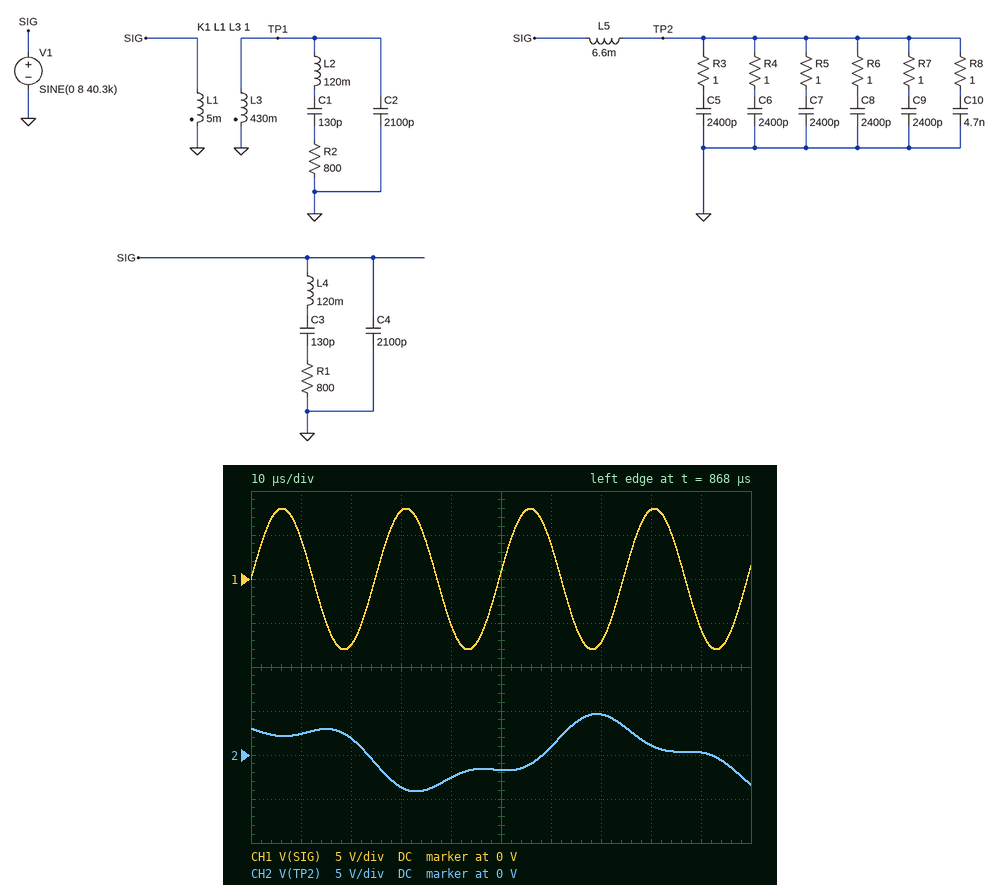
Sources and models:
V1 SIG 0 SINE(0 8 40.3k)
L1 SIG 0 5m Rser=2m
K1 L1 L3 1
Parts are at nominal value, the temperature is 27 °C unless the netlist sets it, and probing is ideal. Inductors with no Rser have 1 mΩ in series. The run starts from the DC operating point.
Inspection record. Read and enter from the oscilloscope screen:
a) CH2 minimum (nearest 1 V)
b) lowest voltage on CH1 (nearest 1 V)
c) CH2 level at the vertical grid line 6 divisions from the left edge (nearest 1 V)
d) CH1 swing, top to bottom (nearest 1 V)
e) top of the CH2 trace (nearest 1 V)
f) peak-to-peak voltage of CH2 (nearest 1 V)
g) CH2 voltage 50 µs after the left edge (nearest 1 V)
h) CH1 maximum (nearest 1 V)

-4 V
-8 V
1 V
16 V
5 V
9 V
-2 V
8 V
